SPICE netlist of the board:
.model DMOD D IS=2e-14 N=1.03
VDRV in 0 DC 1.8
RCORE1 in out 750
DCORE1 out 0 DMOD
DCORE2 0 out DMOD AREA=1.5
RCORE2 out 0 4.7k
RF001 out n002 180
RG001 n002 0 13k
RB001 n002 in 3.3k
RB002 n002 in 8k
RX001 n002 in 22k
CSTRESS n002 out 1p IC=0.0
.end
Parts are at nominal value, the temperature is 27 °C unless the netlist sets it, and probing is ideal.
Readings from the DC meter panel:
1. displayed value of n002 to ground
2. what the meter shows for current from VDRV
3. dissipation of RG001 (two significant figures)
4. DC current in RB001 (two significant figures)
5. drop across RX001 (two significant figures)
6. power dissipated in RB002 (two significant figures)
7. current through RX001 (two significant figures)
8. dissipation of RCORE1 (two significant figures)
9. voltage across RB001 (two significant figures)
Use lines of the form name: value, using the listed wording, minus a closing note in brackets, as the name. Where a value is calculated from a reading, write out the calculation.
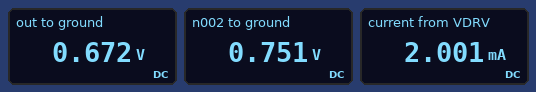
displayed value of n002 to ground: 0.751 V
what the meter shows for current from VDRV: 2.001 mA
dissipation of RG001: (751 mV)^2 / 13 kΩ = 43 µW
DC current in RB001: (1.8 V - 751 mV) / 3.3 kΩ = 320 µA
drop across RX001: 1.8 V - 751 mV = 1.0 V
power dissipated in RB002: (1.8 V - 751 mV)^2 / 8 kΩ = 140 µW
current through RX001: (1.8 V - 751 mV) / 22 kΩ = 48 µA
dissipation of RCORE1: (1.8 V - 672 mV)^2 / 750 Ω = 1.7 mW
voltage across RB001: 1.8 V - 751 mV = 1.0 V
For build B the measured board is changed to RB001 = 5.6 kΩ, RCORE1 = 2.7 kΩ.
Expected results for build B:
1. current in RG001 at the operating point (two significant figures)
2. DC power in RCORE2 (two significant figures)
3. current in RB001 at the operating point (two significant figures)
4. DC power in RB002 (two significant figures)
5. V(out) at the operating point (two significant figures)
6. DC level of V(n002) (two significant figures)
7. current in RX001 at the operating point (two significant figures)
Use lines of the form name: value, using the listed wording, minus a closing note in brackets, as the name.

current in RG001 at the operating point: 54 µA
DC power in RCORE2: 88 µW
current in RB001 at the operating point: 200 µA
DC power in RB002: 150 µW
V(out) at the operating point: 640 mV
DC level of V(n002): 700 mV
current in RX001 at the operating point: 50 µA
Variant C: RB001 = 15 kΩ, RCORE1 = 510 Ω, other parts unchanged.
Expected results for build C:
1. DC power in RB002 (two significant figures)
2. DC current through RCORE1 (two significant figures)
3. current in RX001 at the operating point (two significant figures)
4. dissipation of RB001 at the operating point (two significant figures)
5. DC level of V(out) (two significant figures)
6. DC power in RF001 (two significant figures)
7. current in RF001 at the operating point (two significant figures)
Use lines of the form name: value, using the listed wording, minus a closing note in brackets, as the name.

DC power in RB002: 150 µW
DC current through RCORE1: 2.2 mA
current in RX001 at the operating point: 49 µA
dissipation of RB001 at the operating point: 79 µW
DC level of V(out): 680 mV
DC power in RF001: 7.4 µW
current in RF001 at the operating point: 200 µA
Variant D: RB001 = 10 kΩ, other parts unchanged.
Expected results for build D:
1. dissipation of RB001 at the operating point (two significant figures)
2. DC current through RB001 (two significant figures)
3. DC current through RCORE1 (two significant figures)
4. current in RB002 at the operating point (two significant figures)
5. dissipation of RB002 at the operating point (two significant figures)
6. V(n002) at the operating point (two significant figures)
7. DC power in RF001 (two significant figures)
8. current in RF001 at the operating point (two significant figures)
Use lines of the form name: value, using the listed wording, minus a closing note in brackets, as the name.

dissipation of RB001 at the operating point: 120 µW
DC current through RB001: 110 µA
DC current through RCORE1: 1.5 mA
current in RB002 at the operating point: 140 µA
dissipation of RB002 at the operating point: 150 µW
V(n002) at the operating point: 710 mV
DC power in RF001: 10 µW
current in RF001 at the operating point: 240 µA
